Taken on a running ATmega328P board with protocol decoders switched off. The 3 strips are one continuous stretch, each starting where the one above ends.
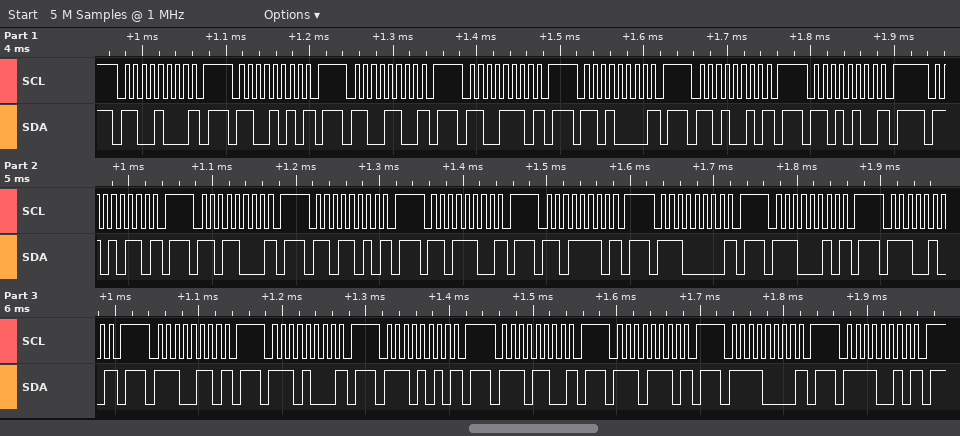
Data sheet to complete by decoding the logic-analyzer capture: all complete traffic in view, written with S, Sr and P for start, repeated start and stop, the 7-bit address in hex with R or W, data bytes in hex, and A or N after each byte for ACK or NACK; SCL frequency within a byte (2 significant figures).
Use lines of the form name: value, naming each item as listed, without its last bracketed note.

all complete traffic in view, written with S, Sr and P for start, repeated start and stop, the 7-bit address in hex with R or W, data bytes in hex, and A or N after each byte for ACK or NACK: S 64W N P S 65W N P S 66W N P S 67W N P S 68W N P S 69W N P S 6AW N P S 6BW N P S 6CW N P S 6DW N P S 6EW N P S 6FW N P S 70W N P S 71W N P S 72W N P S 73W N P S 74W N P S 75W N P S 76W N P S 77W N P S 78W N P S 79W N P
SCL frequency within a byte: 100 kHz
